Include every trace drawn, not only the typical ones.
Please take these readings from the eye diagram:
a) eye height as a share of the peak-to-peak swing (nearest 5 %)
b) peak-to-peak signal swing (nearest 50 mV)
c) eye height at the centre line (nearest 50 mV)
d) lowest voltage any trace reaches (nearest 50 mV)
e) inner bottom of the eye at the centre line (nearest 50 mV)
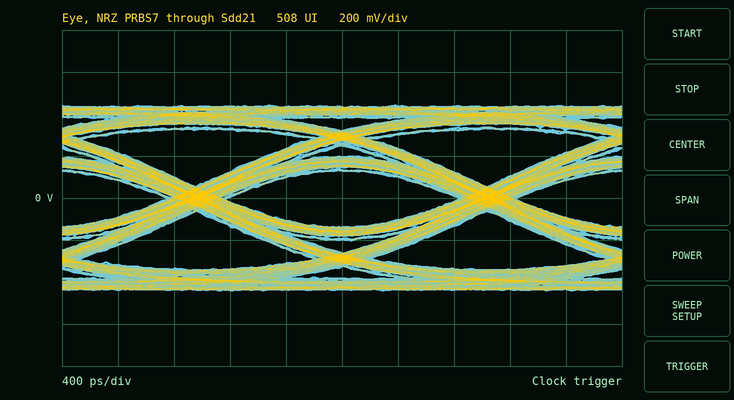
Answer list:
30 %
900 mV
250 mV
-450 mV
-150 mV
